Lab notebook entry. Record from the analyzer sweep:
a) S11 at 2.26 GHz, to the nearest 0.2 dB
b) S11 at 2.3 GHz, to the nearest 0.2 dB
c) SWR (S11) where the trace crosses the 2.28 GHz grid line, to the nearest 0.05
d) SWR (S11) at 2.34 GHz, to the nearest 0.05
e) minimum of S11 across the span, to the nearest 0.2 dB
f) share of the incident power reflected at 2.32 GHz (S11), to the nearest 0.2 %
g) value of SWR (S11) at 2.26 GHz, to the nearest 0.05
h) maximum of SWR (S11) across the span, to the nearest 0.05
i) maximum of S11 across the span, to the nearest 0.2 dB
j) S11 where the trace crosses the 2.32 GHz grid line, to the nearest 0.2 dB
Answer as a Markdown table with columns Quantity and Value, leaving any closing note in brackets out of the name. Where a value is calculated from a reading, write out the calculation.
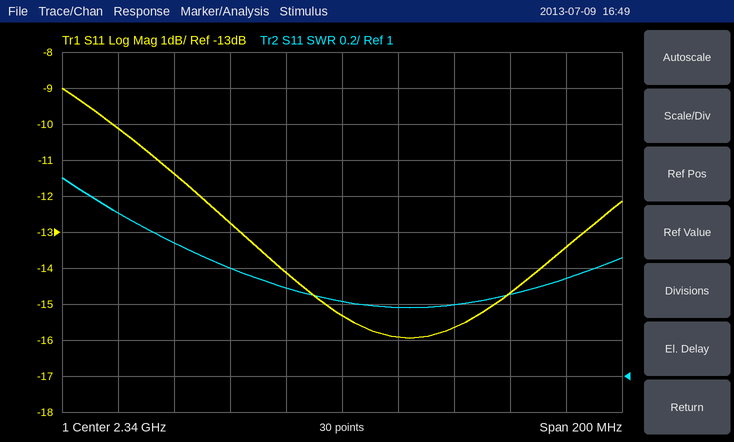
| Quantity | Value |
|---|---|
| S11 at 2.26 GHz, to the nearest 0.2 dB | -10.2 dB |
| S11 at 2.3 GHz, to the nearest 0.2 dB | -12.8 dB |
| SWR (S11) where the trace crosses the 2.28 GHz grid line, to the nearest 0.05 | 1.75 |
| SWR (S11) at 2.34 GHz, to the nearest 0.05 | 1.40 |
| minimum of S11 across the span, to the nearest 0.2 dB | -16.0 dB |
| share of the incident power reflected at 2.32 GHz (S11), to the nearest 0.2 % | 10^(-14.2/10) ≈ 3.8 % |
| value of SWR (S11) at 2.26 GHz, to the nearest 0.05 | 1.90 |
| maximum of SWR (S11) across the span, to the nearest 0.05 | 2.10 |
| maximum of S11 across the span, to the nearest 0.2 dB | -9.0 dB |
| S11 where the trace crosses the 2.32 GHz grid line, to the nearest 0.2 dB | -14.2 dB |
